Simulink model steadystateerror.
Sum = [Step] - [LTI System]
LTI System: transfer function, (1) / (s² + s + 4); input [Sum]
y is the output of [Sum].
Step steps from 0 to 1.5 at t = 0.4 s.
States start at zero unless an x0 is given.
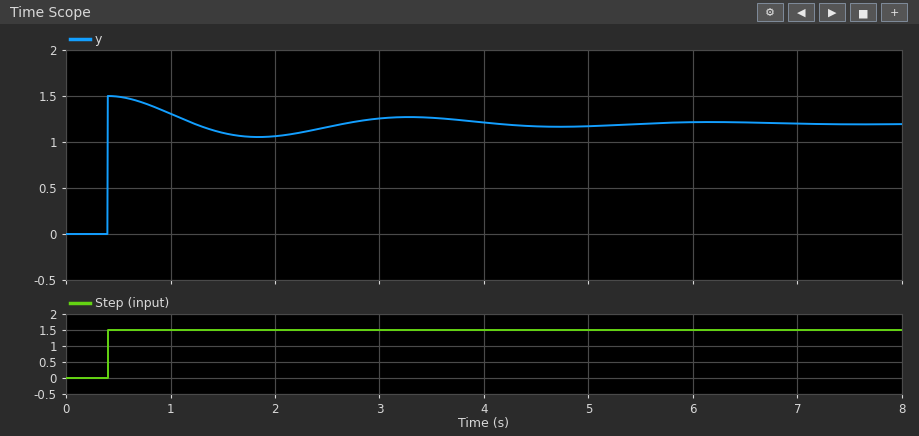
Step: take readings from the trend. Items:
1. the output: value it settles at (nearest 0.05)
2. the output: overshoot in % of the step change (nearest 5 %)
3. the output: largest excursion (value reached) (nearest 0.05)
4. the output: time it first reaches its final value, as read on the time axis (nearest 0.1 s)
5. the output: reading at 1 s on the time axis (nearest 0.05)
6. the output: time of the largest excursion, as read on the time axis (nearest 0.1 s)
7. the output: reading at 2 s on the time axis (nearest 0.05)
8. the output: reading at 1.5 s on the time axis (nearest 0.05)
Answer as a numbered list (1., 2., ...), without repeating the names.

1. 1.20
2. 25 %
3. 1.50
4. 0.4 s
5. 1.30
6. 0.4 s
7. 1.05
8. 1.10
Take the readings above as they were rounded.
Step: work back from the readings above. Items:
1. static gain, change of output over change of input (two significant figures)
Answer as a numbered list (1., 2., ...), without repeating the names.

1. 0.80
